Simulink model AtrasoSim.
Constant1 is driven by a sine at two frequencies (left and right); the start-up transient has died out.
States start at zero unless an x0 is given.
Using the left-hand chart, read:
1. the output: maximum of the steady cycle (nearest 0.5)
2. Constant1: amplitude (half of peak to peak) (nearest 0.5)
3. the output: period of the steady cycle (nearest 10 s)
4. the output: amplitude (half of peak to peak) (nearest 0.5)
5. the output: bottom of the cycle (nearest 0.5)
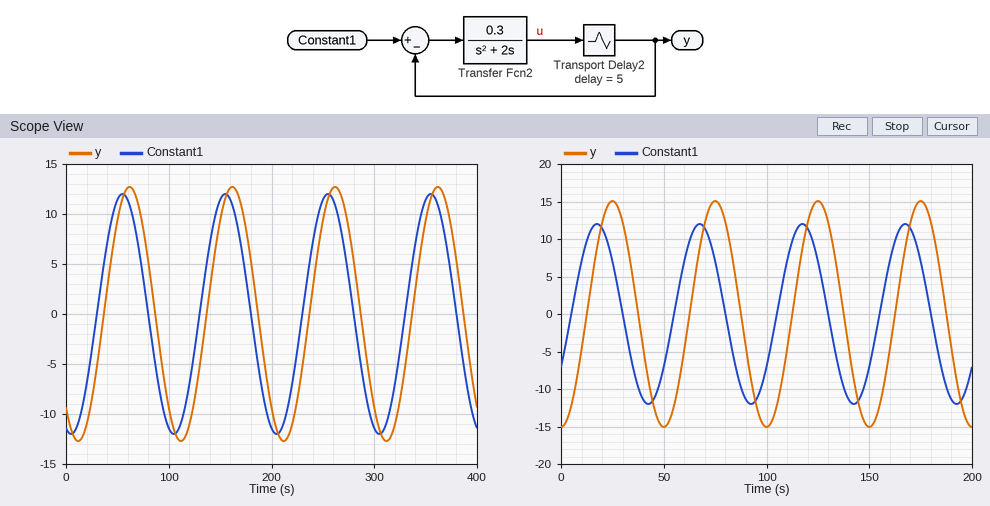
12.5
12.0
100 s
12.5
-12.5
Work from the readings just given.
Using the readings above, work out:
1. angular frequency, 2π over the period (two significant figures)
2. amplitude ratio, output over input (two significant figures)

0.063 rad/s
1.0
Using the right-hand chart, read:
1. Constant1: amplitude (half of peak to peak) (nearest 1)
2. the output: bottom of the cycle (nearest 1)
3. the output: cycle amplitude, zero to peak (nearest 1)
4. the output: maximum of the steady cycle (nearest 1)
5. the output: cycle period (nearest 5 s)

12
-15
15
15
50 s
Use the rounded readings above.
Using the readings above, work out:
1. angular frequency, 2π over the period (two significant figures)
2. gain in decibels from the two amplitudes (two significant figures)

0.13 rad/s
1.9 dB
